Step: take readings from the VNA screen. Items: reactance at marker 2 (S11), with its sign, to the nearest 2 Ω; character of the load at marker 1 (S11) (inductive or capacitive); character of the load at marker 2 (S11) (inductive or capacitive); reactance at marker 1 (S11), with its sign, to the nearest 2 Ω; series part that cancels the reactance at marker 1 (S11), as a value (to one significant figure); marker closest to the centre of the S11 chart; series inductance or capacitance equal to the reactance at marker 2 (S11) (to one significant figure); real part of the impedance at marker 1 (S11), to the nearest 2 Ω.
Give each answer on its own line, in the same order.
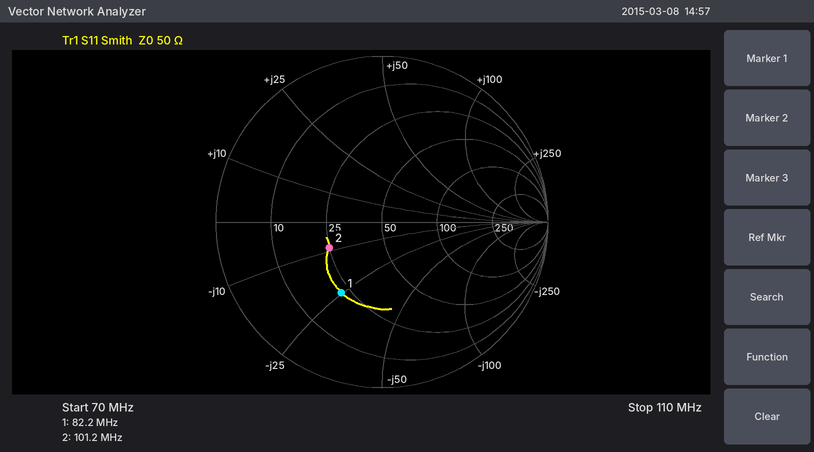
-8 Ω
capacitive
capacitive
-24 Ω
50 nH
marker 2
200 pF
22 Ω
